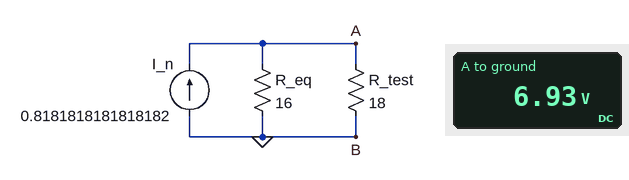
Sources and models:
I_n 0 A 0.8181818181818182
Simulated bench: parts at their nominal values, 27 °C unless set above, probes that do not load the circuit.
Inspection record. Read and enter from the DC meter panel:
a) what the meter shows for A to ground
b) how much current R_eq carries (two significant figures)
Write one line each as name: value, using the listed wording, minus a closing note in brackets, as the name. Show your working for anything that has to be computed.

what the meter shows for A to ground: 6.93 V
how much current R_eq carries: (6.93 V) / 16 Ω = 430 mA
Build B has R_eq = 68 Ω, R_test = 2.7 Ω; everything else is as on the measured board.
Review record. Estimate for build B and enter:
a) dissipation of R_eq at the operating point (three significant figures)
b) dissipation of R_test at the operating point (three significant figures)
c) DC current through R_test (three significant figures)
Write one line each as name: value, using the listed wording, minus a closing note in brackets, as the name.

dissipation of R_eq at the operating point: 66.4 mW
dissipation of R_test at the operating point: 1.67 W
DC current through R_test: 787 mA
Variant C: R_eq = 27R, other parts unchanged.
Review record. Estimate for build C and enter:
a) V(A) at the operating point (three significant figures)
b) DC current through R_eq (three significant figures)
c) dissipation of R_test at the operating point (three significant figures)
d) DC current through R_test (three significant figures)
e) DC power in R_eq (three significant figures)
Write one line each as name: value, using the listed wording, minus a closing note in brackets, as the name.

V(A) at the operating point: 8.84 V
DC current through R_eq: 327 mA
dissipation of R_test at the operating point: 4.34 W
DC current through R_test: 491 mA
DC power in R_eq: 2.89 W
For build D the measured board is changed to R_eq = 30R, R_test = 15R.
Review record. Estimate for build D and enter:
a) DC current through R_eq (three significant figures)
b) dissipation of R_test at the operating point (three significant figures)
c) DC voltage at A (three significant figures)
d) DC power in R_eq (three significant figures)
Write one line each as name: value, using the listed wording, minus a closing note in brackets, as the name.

DC current through R_eq: 273 mA
dissipation of R_test at the operating point: 4.46 W
DC voltage at A: 8.18 V
DC power in R_eq: 2.23 W
